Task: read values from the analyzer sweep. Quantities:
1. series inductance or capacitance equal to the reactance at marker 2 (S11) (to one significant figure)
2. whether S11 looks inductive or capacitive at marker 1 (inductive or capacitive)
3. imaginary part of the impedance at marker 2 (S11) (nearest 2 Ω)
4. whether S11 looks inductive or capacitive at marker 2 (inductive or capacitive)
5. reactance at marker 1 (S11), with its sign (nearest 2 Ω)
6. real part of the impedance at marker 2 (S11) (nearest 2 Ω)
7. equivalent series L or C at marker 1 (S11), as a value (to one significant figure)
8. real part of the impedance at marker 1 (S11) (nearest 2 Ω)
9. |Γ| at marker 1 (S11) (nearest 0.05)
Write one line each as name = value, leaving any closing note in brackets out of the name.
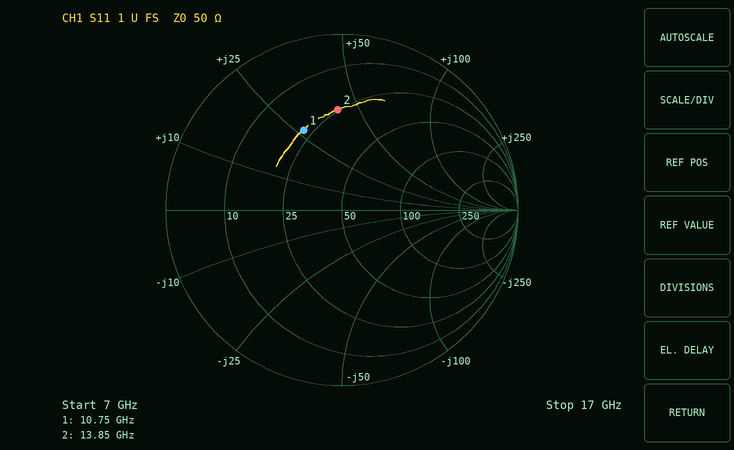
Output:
series inductance or capacitance equal to the reactance at marker 2 (S11) = 500 pH
whether S11 looks inductive or capacitive at marker 1 = inductive
imaginary part of the impedance at marker 2 (S11) = +42 Ω
whether S11 looks inductive or capacitive at marker 2 = inductive
reactance at marker 1 (S11), with its sign = +26 Ω
real part of the impedance at marker 2 (S11) = 24 Ω
equivalent series L or C at marker 1 (S11), as a value = 400 pH
real part of the impedance at marker 1 (S11) = 22 Ω
|Γ| at marker 1 (S11) = 0.50
